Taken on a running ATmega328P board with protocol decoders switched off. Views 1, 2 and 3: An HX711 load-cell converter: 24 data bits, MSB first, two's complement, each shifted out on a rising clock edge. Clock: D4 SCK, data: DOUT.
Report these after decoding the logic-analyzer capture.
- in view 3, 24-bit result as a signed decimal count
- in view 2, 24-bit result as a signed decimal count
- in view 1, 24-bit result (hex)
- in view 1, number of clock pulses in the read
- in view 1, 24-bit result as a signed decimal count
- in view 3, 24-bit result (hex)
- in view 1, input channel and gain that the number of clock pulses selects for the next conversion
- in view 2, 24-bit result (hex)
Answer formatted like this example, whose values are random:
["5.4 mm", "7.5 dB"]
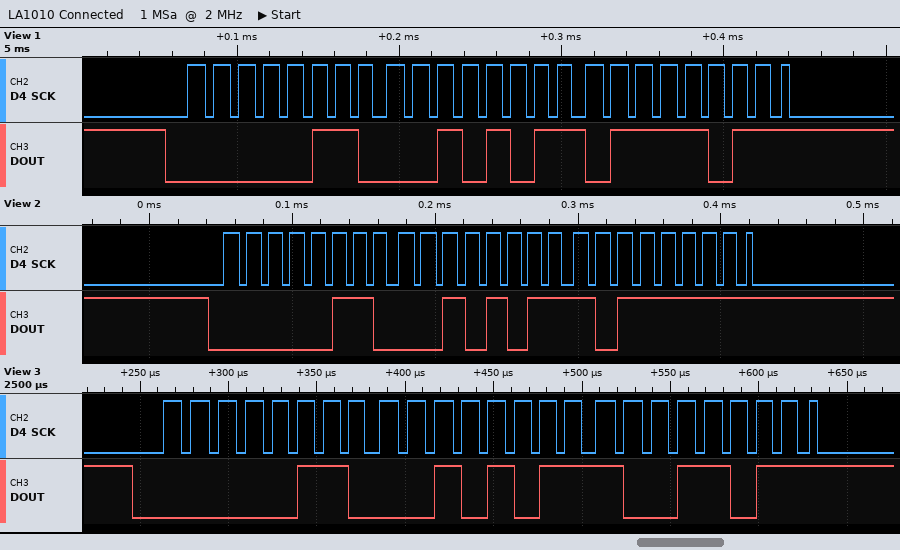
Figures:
["404379", "404415", "0x062B7B", "25", "404347", "0x062B9B", "channel A, gain 128", "0x062BBF"]
